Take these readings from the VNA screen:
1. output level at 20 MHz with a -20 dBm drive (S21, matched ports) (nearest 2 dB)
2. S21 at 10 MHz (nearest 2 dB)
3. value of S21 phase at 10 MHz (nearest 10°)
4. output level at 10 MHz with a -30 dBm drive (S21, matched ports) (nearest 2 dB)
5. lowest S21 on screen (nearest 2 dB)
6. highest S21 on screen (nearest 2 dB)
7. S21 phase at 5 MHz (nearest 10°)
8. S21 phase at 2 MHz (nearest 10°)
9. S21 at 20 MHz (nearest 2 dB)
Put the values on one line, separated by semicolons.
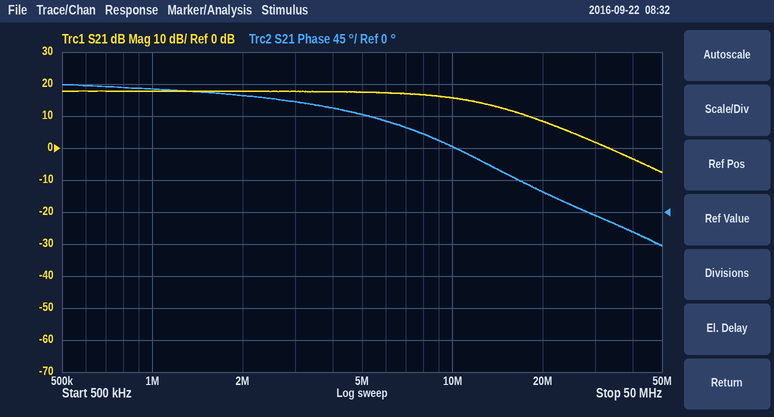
-12 dBm; 16 dB; 90°; -14 dBm; -8 dB; 18 dB; 140°; 160°; 8 dB
